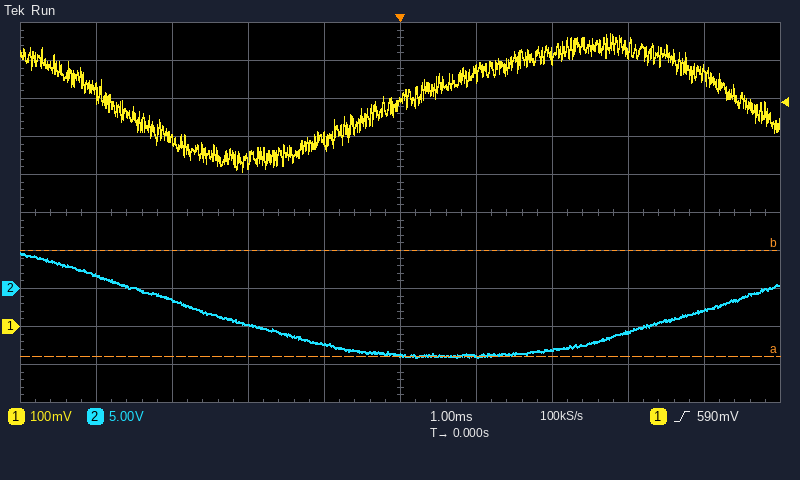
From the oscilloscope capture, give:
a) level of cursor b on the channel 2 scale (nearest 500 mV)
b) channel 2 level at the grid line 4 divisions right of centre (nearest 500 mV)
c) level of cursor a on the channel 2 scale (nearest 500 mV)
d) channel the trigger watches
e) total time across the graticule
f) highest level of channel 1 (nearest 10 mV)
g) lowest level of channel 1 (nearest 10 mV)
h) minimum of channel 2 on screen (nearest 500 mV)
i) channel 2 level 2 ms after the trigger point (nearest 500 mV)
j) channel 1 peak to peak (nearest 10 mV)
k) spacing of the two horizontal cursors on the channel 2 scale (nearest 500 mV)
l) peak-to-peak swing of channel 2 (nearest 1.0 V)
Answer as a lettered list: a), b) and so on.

a) 5.0 V
b) -3.0 V
c) -9.0 V
d) channel 1
e) 10 ms
f) 770 mV
g) 410 mV
h) -9.0 V
i) -8.0 V
j) 360 mV
k) 14.0 V
l) 14.0 V
